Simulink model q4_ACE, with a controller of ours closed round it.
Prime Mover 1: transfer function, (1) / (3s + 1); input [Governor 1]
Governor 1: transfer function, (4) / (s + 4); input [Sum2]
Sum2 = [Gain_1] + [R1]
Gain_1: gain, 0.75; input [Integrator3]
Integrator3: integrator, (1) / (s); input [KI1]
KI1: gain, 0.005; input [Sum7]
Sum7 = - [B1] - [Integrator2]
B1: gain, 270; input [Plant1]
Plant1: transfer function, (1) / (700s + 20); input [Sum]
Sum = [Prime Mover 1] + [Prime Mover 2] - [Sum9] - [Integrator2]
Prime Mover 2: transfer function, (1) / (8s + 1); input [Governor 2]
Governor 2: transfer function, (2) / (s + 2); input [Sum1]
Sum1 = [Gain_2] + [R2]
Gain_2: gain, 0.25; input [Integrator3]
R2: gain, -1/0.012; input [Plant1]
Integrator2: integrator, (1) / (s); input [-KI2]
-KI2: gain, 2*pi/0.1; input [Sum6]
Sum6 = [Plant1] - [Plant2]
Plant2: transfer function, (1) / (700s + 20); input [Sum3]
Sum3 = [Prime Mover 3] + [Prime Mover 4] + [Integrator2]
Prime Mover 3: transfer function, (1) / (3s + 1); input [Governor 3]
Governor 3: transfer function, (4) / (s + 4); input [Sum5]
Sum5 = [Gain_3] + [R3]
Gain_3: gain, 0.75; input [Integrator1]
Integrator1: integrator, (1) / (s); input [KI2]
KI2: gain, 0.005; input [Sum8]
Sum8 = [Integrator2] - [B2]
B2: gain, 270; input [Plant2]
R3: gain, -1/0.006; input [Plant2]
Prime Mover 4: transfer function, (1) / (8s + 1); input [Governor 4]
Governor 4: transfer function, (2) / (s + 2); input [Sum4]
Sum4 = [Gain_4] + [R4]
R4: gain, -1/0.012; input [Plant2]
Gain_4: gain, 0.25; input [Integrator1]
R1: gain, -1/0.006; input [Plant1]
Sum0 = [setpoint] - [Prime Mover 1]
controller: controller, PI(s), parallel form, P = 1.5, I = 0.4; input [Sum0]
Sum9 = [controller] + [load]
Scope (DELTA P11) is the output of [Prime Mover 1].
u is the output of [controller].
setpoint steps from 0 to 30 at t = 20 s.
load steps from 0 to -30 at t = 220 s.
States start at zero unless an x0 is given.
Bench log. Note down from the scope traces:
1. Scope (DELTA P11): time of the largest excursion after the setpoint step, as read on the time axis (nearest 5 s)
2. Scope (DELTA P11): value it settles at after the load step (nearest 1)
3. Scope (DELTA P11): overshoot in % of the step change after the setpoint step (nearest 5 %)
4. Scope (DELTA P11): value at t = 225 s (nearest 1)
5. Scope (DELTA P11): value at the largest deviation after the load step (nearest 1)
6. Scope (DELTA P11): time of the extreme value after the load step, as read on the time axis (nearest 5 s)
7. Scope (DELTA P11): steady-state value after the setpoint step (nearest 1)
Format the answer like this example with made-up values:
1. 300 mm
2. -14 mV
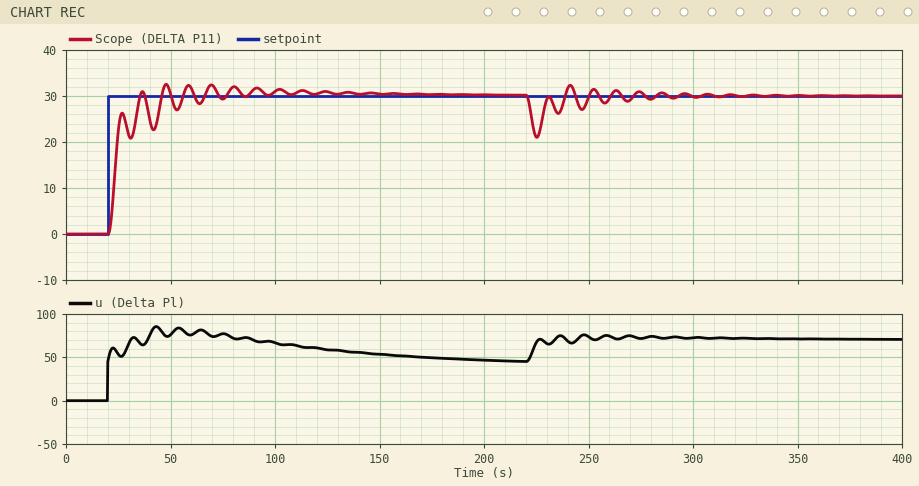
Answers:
1. 50 s
2. 30
3. 10 %
4. 21
5. 21
6. 225 s
7. 30
